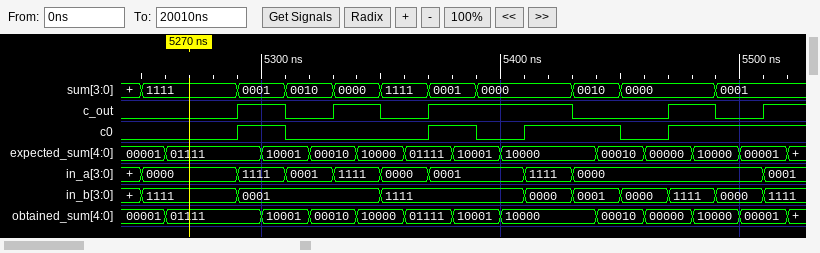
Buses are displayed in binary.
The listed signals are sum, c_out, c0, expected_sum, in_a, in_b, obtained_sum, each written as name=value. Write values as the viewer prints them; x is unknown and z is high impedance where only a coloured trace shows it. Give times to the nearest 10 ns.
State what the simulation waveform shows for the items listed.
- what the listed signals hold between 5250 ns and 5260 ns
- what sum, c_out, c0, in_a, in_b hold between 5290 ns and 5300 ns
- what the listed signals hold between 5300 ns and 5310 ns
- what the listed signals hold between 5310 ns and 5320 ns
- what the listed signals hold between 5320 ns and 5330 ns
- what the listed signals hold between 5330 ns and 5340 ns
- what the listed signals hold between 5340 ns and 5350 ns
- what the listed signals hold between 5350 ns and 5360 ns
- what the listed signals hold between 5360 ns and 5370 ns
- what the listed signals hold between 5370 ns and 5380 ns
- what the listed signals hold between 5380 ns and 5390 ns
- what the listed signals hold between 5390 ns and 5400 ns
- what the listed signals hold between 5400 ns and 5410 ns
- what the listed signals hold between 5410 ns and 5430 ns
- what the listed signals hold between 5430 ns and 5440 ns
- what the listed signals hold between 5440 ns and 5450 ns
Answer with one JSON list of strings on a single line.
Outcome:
["sum=1111, c_out=0, c0=0, expected_sum=00001, in_a=0000, in_b=1111, obtained_sum=00001", "sum=0001, c_out=1, c0=1, in_a=1111, in_b=0001", "sum=0001, c_out=1, c0=1, expected_sum=10001, in_a=1111, in_b=0001, obtained_sum=10001", "sum=0010, c_out=0, c0=0, expected_sum=10001, in_a=0001, in_b=0001, obtained_sum=10001", "sum=0010, c_out=0, c0=0, expected_sum=00010, in_a=0001, in_b=0001, obtained_sum=00010", "sum=0000, c_out=1, c0=0, expected_sum=00010, in_a=1111, in_b=0001, obtained_sum=00010", "sum=0000, c_out=1, c0=0, expected_sum=10000, in_a=1111, in_b=0001, obtained_sum=10000", "sum=1111, c_out=0, c0=0, expected_sum=10000, in_a=0000, in_b=1111, obtained_sum=10000", "sum=1111, c_out=0, c0=0, expected_sum=01111, in_a=0000, in_b=1111, obtained_sum=01111", "sum=0001, c_out=1, c0=1, expected_sum=01111, in_a=0001, in_b=1111, obtained_sum=01111", "sum=0001, c_out=1, c0=1, expected_sum=10001, in_a=0001, in_b=1111, obtained_sum=10001", "sum=0000, c_out=1, c0=0, expected_sum=10001, in_a=0001, in_b=1111, obtained_sum=10001", "sum=0000, c_out=1, c0=0, expected_sum=10000, in_a=0001, in_b=1111, obtained_sum=10000", "sum=0000, c_out=1, c0=1, expected_sum=10000, in_a=1111, in_b=0000, obtained_sum=10000", "sum=0010, c_out=0, c0=1, expected_sum=10000, in_a=0000, in_b=0001, obtained_sum=10000", "sum=0010, c_out=0, c0=1, expected_sum=00010, in_a=0000, in_b=0001, obtained_sum=00010"]
